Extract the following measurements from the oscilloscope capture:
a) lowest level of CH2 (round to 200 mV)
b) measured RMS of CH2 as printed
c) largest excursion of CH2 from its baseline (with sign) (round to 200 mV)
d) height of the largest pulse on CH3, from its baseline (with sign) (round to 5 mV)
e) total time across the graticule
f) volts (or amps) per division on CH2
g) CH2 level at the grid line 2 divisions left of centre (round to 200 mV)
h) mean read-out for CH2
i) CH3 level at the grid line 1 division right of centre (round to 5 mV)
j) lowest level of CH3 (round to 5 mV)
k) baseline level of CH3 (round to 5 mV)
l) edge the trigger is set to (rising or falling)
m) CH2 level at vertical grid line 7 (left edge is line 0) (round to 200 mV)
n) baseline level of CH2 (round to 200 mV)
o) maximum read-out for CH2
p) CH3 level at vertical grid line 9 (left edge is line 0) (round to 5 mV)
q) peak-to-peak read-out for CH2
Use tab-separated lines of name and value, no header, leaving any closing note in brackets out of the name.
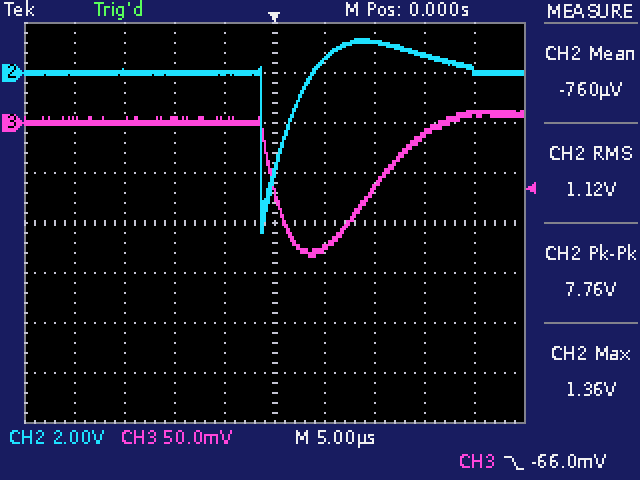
lowest level of CH2	-6.4 V
measured RMS of CH2 as printed	1.12 V
largest excursion of CH2 from its baseline (with sign)	-6.4 V
height of the largest pulse on CH3, from its baseline (with sign)	-135 mV
total time across the graticule	50 µs
volts (or amps) per division on CH2	2 V
CH2 level at the grid line 2 divisions left of centre	0.0 V
mean read-out for CH2	-760 µV
CH3 level at the grid line 1 division right of centre	-125 mV
lowest level of CH3	-135 mV
baseline level of CH3	0 mV
edge the trigger is set to	falling
CH2 level at vertical grid line 7 (left edge is line 0)	1.2 V
baseline level of CH2	0.0 V
maximum read-out for CH2	1.36 V
CH3 level at vertical grid line 9 (left edge is line 0)	10 mV
peak-to-peak read-out for CH2	7.76 V
